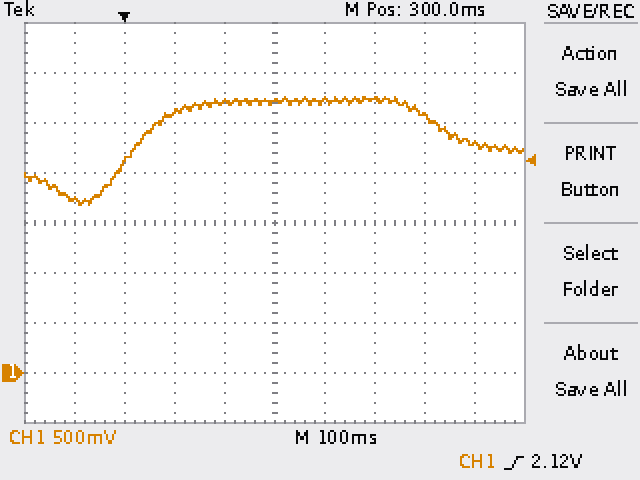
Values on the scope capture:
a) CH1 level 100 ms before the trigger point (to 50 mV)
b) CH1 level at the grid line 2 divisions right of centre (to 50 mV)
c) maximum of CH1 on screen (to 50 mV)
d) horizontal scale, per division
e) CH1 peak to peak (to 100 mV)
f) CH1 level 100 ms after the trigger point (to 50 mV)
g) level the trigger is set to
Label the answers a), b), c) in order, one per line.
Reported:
a) 1.75 V
b) 2.75 V
c) 2.75 V
d) 100 ms
e) 1.10 V
f) 2.60 V
g) 2.12 V
